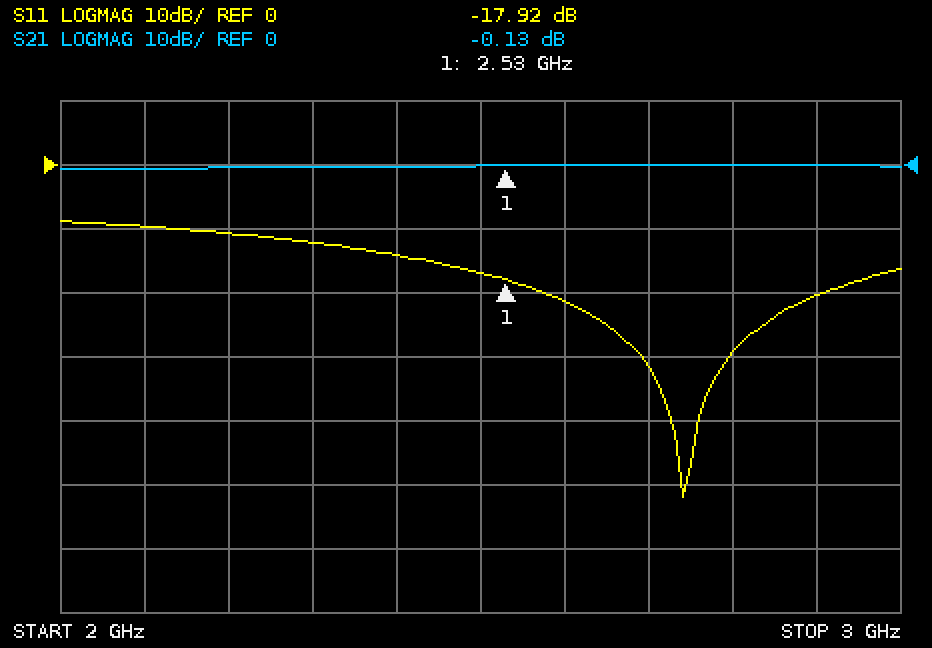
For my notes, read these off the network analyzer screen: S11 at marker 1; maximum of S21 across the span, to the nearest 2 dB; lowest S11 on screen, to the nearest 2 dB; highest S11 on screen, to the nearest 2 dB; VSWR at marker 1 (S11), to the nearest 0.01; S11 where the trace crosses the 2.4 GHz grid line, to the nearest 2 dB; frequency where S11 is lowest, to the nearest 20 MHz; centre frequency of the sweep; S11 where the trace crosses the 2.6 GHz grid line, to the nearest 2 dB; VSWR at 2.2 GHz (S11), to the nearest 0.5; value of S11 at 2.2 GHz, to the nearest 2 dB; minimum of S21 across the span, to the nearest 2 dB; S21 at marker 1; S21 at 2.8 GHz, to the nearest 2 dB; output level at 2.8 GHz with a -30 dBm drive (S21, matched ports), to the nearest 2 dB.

-17.92 dB
0 dB
-52 dB
-8 dB
1.29
-14 dB
2.74 GHz
2.5 GHz
-22 dB
2.0
-10 dB
0 dB
-0.13 dB
0 dB
-30 dBm
